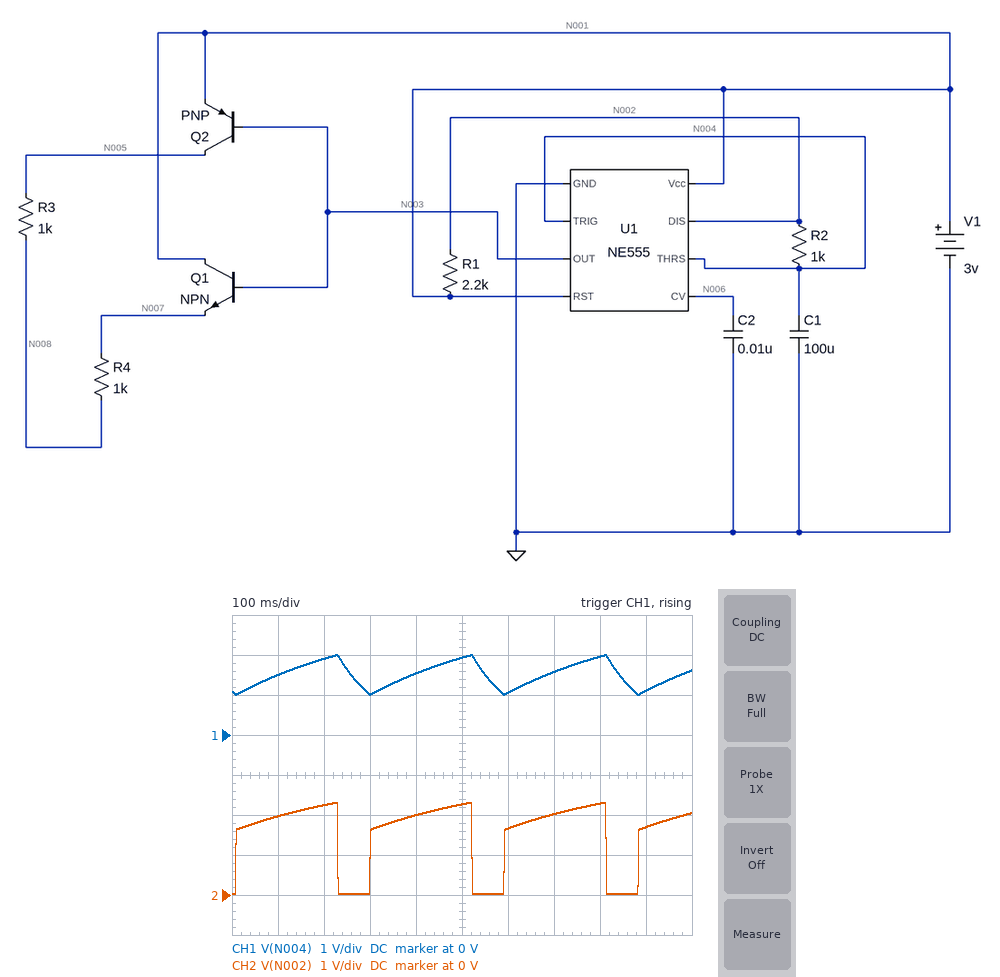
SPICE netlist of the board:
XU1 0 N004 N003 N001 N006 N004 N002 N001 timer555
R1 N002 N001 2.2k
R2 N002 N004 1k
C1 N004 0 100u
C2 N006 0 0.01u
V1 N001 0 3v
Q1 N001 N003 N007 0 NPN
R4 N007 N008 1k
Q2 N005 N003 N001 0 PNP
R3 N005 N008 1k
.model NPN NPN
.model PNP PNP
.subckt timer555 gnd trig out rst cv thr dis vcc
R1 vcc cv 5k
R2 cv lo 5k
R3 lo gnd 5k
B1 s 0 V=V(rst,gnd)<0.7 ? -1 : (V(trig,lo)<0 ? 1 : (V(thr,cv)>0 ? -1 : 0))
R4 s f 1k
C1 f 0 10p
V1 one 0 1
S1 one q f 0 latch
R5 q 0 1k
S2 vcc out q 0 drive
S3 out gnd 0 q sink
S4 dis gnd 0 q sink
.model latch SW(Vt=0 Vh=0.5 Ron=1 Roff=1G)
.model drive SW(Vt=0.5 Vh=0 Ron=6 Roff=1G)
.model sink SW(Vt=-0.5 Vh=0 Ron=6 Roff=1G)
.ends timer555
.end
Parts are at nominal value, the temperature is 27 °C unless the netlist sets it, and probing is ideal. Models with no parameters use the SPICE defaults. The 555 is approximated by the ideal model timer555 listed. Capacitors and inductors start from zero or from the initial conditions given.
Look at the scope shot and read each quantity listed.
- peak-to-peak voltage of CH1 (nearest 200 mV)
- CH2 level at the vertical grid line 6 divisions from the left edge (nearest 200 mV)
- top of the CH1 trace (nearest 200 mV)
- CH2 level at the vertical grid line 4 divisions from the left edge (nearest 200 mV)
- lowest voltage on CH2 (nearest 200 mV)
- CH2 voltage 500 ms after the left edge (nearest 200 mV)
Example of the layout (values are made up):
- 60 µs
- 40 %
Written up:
- 1.0 V
- 1.6 V
- 2.0 V
- 2.0 V
- 0 V
- 2.2 V
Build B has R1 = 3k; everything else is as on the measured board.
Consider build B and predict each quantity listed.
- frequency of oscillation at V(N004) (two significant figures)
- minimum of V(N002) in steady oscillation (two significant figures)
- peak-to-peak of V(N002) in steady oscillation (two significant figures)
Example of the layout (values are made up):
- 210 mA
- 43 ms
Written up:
- 2.9 Hz
- 12 mV
- 2.2 V
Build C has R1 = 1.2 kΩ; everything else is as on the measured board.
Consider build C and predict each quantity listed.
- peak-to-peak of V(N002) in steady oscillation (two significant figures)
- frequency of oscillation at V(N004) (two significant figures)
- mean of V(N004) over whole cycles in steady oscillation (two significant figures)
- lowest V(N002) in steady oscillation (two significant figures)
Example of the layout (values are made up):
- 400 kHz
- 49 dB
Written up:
- 2.4 V
- 4.5 Hz
- 1.5 V
- 21 mV
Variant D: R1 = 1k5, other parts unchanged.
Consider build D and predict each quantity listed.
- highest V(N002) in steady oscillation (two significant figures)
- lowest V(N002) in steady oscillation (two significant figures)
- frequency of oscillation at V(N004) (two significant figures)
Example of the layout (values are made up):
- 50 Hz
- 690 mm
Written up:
- 2.4 V
- 18 mV
- 4.1 Hz
